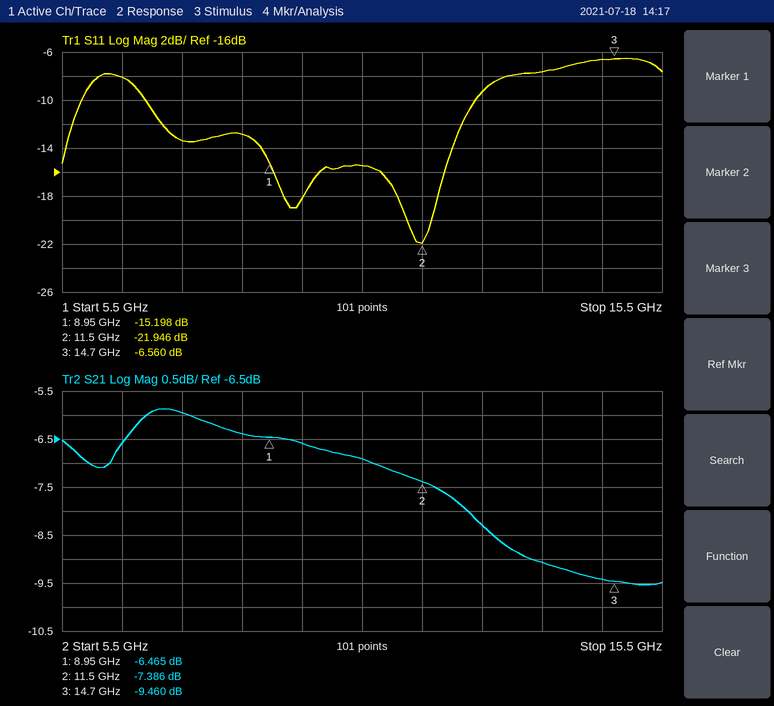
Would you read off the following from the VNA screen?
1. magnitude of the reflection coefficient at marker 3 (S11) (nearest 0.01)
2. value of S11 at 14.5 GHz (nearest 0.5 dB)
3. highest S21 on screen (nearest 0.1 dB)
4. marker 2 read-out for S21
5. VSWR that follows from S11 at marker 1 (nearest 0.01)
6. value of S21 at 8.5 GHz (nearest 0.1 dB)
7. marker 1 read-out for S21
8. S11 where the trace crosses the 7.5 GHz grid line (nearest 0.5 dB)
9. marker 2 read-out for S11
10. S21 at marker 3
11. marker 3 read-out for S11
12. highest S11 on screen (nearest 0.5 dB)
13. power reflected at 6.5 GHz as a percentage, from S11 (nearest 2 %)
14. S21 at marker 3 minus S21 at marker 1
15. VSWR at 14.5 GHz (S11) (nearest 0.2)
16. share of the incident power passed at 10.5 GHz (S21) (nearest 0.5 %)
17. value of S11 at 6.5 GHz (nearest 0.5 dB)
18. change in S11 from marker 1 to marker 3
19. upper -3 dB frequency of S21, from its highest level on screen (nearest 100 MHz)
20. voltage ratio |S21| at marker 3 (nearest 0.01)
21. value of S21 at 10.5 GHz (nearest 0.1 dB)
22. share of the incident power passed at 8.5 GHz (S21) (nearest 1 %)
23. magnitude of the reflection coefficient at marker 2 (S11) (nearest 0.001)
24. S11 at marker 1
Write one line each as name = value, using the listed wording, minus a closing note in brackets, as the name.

magnitude of the reflection coefficient at marker 3 (S11) = 0.47
value of S11 at 14.5 GHz = -6.5 dB
highest S21 on screen = -5.9 dB
marker 2 read-out for S21 = -7.386 dB
VSWR that follows from S11 at marker 1 = 1.42
value of S21 at 8.5 GHz = -6.4 dB
marker 1 read-out for S21 = -6.465 dB
S11 where the trace crosses the 7.5 GHz grid line = -13.5 dB
marker 2 read-out for S11 = -21.946 dB
S21 at marker 3 = -9.460 dB
marker 3 read-out for S11 = -6.560 dB
highest S11 on screen = -6.5 dB
power reflected at 6.5 GHz as a percentage, from S11 = 16 %
S21 at marker 3 minus S21 at marker 1 = -2.995 dB
VSWR at 14.5 GHz (S11) = 2.8
share of the incident power passed at 10.5 GHz (S21) = 20.5 %
value of S11 at 6.5 GHz = -8.0 dB
change in S11 from marker 1 to marker 3 = 8.638 dB
upper -3 dB frequency of S21, from its highest level on screen = 13.1 GHz
voltage ratio |S21| at marker 3 = 0.34
value of S21 at 10.5 GHz = -6.9 dB
share of the incident power passed at 8.5 GHz (S21) = 23 %
magnitude of the reflection coefficient at marker 2 (S11) = 0.080
S11 at marker 1 = -15.198 dB
